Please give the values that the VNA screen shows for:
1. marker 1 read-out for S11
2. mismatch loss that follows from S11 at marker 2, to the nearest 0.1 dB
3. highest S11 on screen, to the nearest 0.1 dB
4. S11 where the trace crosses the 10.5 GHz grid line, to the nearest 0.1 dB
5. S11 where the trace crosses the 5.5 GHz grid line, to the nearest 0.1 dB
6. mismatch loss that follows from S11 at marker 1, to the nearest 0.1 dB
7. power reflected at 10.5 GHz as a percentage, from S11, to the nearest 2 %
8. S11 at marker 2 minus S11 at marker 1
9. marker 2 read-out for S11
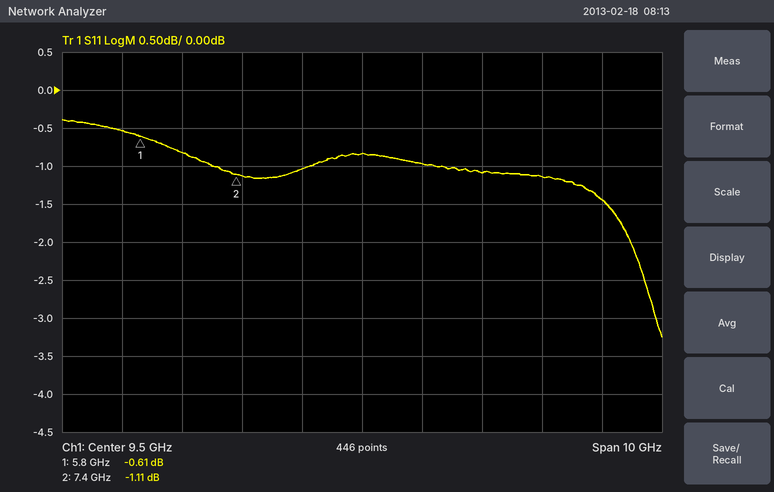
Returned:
-0.61 dB
6.5 dB
-0.4 dB
-1.0 dB
-0.5 dB
8.8 dB
80 %
-0.50 dB
-1.11 dB
